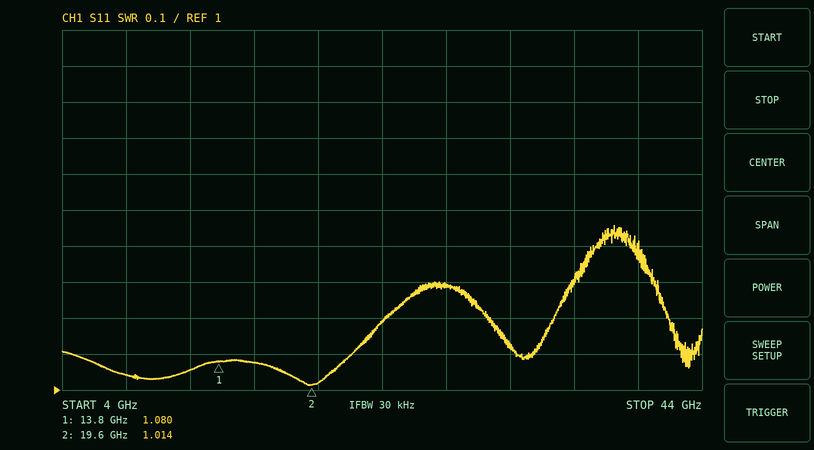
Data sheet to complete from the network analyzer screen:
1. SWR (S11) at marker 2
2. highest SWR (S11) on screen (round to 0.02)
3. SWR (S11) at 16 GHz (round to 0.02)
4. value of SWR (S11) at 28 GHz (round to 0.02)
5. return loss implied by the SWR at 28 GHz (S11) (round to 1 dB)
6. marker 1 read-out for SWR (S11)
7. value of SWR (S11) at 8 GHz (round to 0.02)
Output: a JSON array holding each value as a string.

["1.014", "1.46", "1.08", "1.30", "18 dB", "1.080", "1.04"]
